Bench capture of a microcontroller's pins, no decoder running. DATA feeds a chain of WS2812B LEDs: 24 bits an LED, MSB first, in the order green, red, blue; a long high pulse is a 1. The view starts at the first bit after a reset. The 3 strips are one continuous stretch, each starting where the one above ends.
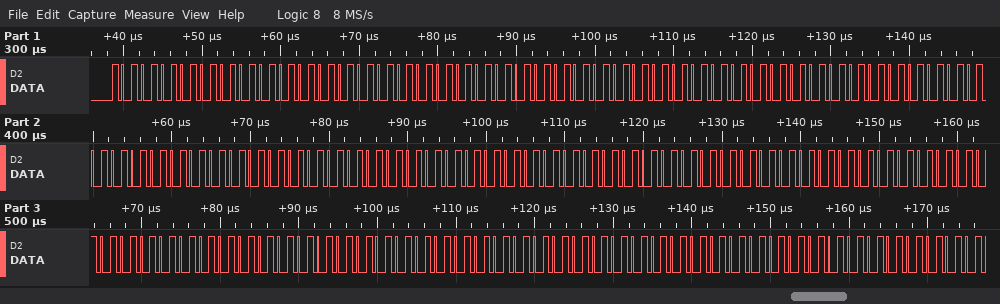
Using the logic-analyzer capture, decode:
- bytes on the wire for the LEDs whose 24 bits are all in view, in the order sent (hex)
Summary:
AA AA AA AA AA AA AA AA AA AA AA AA AA AA AA AA AA AA AA AA AA AA AA AA AA AA AA AA AA AA AA AA AA
